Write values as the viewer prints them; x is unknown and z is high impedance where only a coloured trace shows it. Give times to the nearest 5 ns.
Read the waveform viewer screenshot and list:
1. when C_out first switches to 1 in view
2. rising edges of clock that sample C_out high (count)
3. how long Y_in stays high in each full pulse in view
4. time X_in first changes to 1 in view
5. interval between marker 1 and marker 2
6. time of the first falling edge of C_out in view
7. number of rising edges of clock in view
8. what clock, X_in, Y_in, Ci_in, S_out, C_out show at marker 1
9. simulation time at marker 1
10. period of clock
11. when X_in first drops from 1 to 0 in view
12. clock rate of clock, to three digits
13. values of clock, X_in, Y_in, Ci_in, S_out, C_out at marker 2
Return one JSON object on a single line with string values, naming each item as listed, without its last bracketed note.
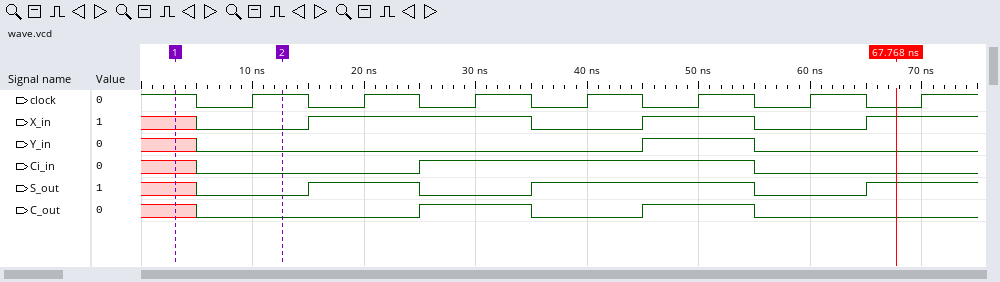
{"when C_out first switches to 1 in view": "25 ns", "rising edges of clock that sample C_out high": "2", "how long Y_in stays high in each full pulse in view": "10 ns", "time X_in first changes to 1 in view": "15 ns", "interval between marker 1 and marker 2": "10 ns", "time of the first falling edge of C_out in view": "35 ns", "number of rising edges of clock in view": "7", "what clock, X_in, Y_in, Ci_in, S_out, C_out show at marker 1": "clock=1, X_in=x, Y_in=x, Ci_in=x, S_out=x, C_out=x", "simulation time at marker 1": "5 ns", "period of clock": "10 ns", "when X_in first drops from 1 to 0 in view": "35 ns", "clock rate of clock, to three digits": "100 MHz", "values of clock, X_in, Y_in, Ci_in, S_out, C_out at marker 2": "clock=1, X_in=0, Y_in=0, Ci_in=0, S_out=0, C_out=0"}
